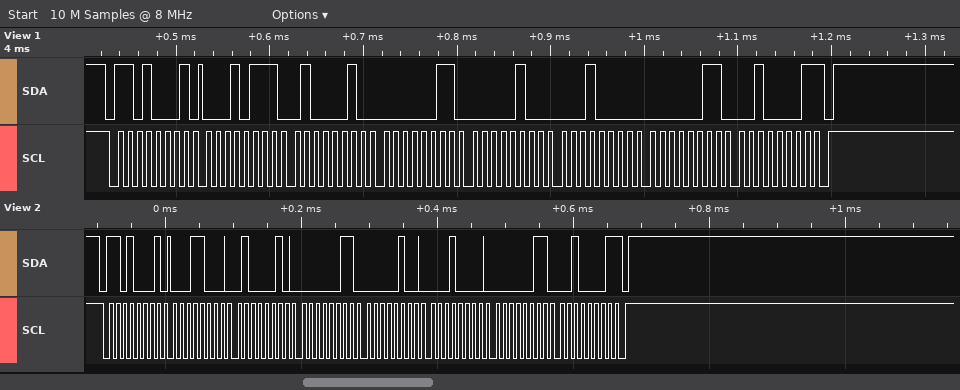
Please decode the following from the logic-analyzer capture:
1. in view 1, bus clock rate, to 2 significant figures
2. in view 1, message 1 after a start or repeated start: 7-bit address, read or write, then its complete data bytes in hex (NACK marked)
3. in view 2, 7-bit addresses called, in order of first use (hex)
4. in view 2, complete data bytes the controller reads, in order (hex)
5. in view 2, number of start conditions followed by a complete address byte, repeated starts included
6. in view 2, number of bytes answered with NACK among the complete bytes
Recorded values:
100 kHz
0x68 read: 17 42 03 04 10 03 21 NACK
0x68
18 42 03 04 10 03 21
1
1
